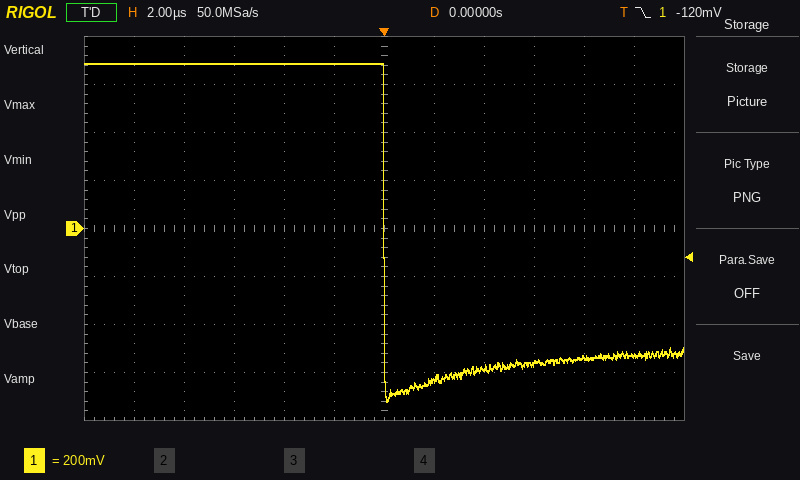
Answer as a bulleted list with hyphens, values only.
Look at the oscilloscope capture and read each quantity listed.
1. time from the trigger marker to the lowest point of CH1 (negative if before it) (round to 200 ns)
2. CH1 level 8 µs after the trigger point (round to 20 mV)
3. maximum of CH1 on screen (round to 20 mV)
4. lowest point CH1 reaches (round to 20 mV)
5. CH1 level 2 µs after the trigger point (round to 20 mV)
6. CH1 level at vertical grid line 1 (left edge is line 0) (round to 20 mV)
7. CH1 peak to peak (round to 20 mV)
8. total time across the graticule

- +200 ns
- -540 mV
- 680 mV
- -720 mV
- -620 mV
- 680 mV
- 1.40 V
- 24 µs
